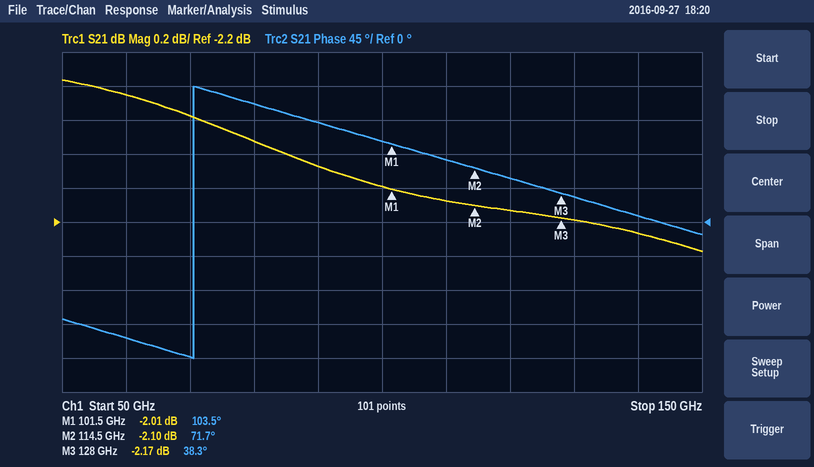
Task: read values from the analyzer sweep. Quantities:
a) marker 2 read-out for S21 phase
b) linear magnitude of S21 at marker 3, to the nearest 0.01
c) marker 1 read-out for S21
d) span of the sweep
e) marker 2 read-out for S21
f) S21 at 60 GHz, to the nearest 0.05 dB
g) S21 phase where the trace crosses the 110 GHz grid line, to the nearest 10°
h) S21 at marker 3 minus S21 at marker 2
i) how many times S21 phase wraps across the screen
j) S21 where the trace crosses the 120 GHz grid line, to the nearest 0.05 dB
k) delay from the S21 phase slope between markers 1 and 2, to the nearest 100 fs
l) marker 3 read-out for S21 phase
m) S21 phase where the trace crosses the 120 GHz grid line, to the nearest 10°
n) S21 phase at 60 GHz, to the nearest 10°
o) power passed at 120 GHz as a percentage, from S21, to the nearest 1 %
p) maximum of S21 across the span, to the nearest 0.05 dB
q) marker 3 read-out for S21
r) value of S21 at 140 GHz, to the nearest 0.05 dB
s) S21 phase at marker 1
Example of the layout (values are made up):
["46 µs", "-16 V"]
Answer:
["71.7°", "0.78", "-2.01 dB", "100 GHz", "-2.10 dB", "-1.45 dB", "80°", "-0.07 dB", "1", "-2.15 dB", "6.8 ps", "38.3°", "60°", "-150°", "61 %", "-1.35 dB", "-2.17 dB", "-2.25 dB", "103.5°"]
